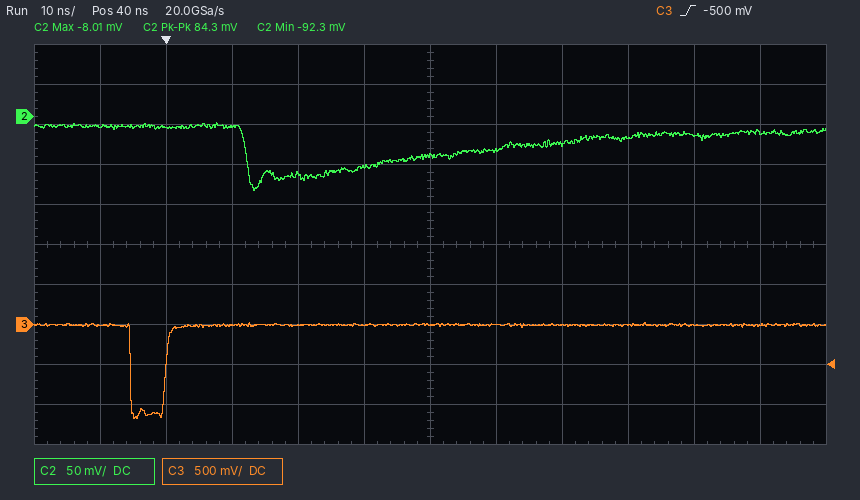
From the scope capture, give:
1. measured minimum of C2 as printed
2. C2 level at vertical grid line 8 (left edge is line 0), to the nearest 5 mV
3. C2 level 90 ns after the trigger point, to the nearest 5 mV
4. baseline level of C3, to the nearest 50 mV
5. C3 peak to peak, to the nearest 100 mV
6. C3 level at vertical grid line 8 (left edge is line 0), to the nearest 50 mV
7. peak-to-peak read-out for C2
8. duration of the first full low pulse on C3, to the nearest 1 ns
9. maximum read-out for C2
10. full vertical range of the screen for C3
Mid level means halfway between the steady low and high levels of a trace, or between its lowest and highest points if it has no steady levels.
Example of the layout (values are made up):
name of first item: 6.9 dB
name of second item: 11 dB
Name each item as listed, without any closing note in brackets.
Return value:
measured minimum of C2 as printed: -92.3 mV
C2 level at vertical grid line 8 (left edge is line 0), to the nearest 5 mV: -35 mV
C2 level 90 ns after the trigger point, to the nearest 5 mV: -20 mV
baseline level of C3, to the nearest 50 mV: 0 mV
C3 peak to peak, to the nearest 100 mV: 1.20 V
C3 level at vertical grid line 8 (left edge is line 0), to the nearest 50 mV: 0 mV
peak-to-peak read-out for C2: 84.3 mV
duration of the first full low pulse on C3, to the nearest 1 ns: 5 ns
maximum read-out for C2: -8.01 mV
full vertical range of the screen for C3: 5 V
